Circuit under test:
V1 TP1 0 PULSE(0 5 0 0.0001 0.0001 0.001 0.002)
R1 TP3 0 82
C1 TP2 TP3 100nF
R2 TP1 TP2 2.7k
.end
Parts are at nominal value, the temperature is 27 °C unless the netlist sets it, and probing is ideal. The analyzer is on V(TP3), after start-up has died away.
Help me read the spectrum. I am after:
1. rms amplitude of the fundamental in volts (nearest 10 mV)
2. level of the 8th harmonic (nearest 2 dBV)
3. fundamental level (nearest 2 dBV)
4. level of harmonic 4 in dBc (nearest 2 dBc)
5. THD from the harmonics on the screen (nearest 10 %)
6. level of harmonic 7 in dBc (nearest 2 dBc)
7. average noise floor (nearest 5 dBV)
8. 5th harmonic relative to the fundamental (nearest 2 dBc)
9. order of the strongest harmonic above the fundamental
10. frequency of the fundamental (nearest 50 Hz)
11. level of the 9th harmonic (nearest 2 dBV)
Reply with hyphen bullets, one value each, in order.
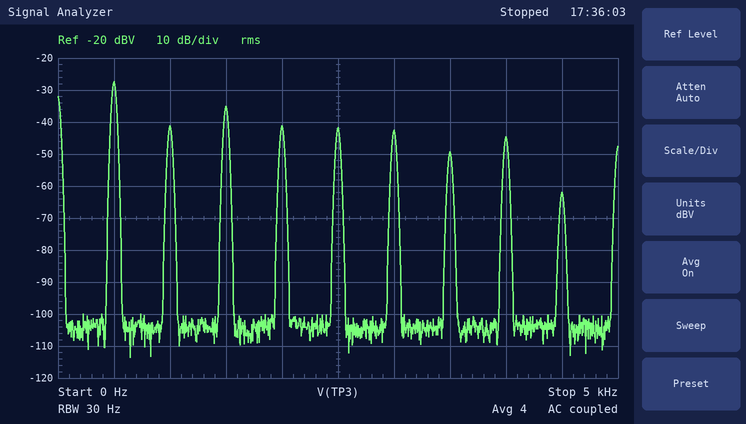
- 40 mV
- -44 dBV
- -28 dBV
- -14 dBc
- 60 %
- -22 dBc
- -105 dBV
- -14 dBc
- 3
- 500 Hz
- -62 dBV
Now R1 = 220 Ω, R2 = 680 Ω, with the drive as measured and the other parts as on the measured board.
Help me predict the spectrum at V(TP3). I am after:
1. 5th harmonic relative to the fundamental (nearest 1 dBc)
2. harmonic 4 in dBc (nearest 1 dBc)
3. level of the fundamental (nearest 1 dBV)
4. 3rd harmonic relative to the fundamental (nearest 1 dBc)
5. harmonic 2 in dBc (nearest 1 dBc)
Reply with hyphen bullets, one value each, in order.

- -8 dBc
- -8 dBc
- -17 dBV
- -3 dBc
- -11 dBc
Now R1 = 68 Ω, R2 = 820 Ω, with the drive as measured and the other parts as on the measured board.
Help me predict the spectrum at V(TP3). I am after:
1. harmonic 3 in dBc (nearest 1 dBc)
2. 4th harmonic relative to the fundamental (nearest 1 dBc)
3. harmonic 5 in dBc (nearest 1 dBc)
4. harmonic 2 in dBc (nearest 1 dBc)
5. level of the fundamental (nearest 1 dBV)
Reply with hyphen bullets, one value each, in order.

- -3 dBc
- -8 dBc
- -8 dBc
- -11 dBc
- -27 dBV
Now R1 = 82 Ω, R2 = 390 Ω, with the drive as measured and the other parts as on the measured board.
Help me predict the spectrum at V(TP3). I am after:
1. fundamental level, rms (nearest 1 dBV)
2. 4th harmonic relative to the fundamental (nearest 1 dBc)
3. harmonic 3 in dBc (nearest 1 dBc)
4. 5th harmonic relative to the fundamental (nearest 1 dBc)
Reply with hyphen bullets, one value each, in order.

- -25 dBV
- -6 dBc
- -2 dBc
- -6 dBc
